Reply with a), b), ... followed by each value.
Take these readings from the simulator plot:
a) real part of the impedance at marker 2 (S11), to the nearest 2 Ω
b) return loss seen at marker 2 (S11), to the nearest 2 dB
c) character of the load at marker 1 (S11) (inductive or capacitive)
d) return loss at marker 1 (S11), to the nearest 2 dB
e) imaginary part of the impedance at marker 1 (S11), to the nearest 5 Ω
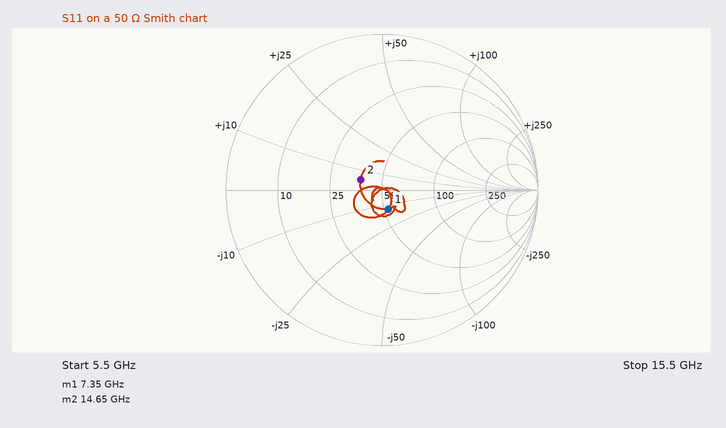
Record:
a) 38 Ω
b) 16 dB
c) capacitive
d) 18 dB
e) -15 Ω
